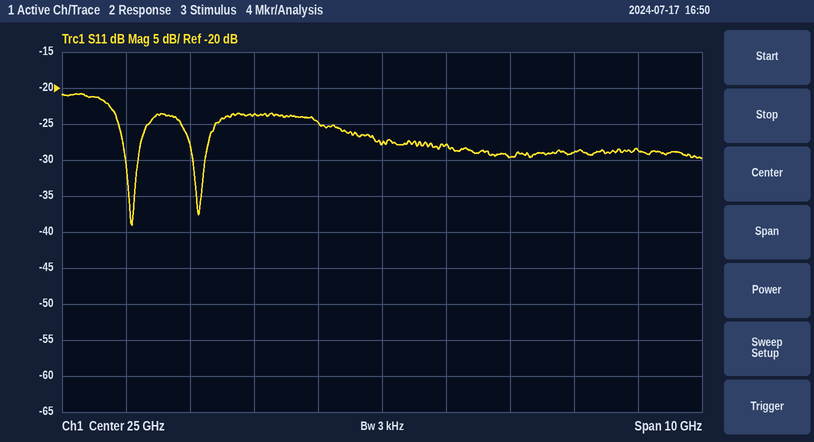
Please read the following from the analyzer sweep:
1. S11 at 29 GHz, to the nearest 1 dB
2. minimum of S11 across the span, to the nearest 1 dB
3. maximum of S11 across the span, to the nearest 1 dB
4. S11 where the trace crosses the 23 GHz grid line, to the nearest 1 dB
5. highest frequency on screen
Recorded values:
-29 dB
-39 dB
-21 dB
-24 dB
30 GHz
